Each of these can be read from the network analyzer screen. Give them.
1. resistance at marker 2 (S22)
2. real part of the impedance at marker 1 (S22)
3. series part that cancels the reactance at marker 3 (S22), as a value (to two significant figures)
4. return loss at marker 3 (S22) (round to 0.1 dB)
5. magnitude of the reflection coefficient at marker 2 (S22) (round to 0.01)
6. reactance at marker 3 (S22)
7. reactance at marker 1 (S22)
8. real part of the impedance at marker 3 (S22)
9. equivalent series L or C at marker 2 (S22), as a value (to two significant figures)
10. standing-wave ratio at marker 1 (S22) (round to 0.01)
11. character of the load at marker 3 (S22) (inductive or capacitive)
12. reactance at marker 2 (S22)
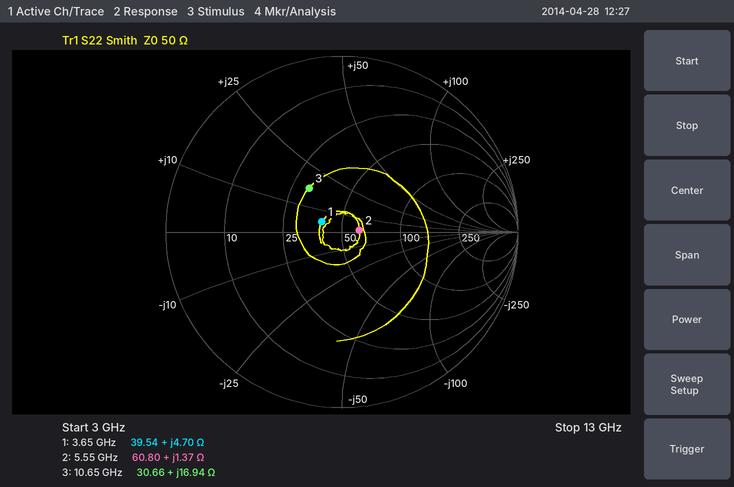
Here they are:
60.80 Ω
39.54 Ω
880 fF
10.1 dB
0.10
+16.94 Ω
+4.70 Ω
30.66 Ω
39 pH
1.29
inductive
+1.37 Ω
